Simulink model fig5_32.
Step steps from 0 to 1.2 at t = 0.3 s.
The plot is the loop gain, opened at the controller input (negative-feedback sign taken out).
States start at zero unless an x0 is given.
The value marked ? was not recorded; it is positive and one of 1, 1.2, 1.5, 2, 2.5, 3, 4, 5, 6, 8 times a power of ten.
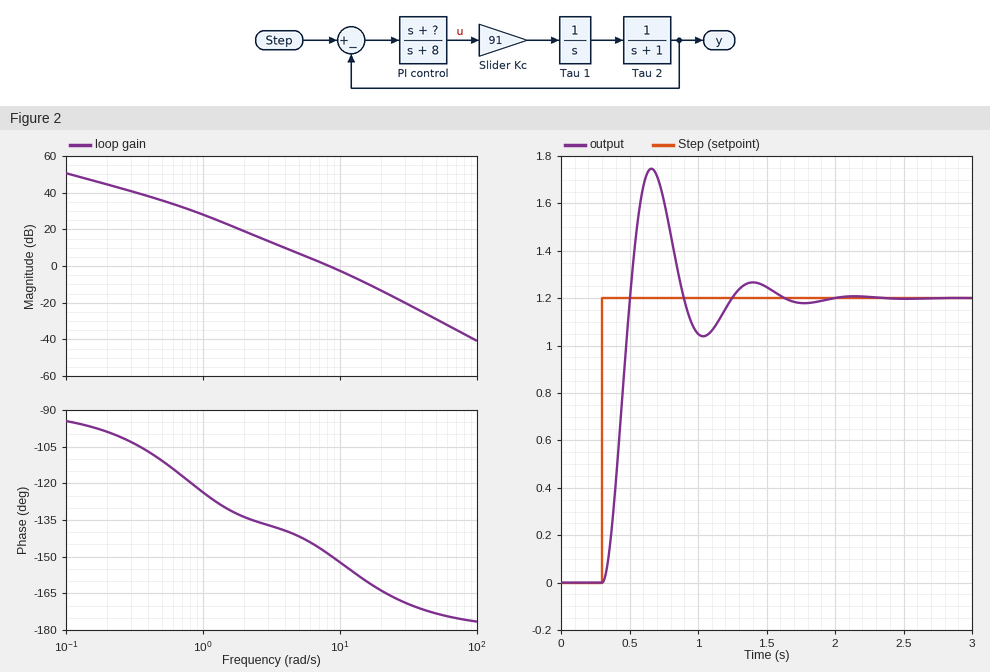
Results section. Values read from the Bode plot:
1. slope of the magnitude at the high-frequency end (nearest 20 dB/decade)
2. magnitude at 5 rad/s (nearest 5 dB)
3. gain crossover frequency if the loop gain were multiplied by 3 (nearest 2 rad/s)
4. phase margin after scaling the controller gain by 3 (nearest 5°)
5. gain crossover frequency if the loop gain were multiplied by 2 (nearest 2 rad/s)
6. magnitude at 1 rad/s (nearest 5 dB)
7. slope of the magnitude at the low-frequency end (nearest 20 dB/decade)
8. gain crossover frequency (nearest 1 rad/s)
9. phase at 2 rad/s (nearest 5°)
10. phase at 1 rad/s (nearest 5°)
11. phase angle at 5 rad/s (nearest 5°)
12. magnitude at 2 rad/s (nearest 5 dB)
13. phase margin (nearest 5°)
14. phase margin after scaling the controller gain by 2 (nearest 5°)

-40 dB/decade
5 dB
16 rad/s
20°
12 rad/s
30 dB
-20 dB/decade
8 rad/s
-135°
-125°
-140°
20 dB
30°
25°
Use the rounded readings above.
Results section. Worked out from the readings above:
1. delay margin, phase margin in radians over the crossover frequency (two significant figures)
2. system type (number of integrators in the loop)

0.065 s
1
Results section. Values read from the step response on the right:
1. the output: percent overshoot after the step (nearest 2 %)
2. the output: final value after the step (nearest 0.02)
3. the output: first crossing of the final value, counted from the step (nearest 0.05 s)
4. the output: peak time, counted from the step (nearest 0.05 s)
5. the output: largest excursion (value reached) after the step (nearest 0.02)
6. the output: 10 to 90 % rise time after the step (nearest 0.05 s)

46 %
1.20
0.20 s
0.35 s
1.74
0.15 s
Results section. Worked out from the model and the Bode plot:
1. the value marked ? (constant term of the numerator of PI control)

3
